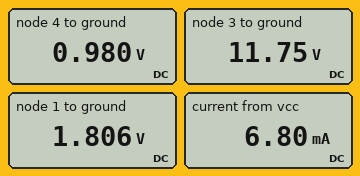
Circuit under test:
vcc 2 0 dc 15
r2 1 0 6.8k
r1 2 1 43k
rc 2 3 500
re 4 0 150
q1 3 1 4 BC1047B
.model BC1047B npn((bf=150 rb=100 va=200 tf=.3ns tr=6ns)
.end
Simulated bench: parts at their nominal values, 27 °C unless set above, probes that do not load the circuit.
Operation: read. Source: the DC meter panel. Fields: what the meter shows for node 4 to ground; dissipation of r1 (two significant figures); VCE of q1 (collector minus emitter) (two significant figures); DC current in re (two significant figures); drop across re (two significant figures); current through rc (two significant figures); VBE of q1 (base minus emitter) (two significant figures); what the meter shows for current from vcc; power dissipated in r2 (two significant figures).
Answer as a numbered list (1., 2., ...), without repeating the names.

1. 0.980 V
2. 4.0 mW
3. 11 V
4. 6.5 mA
5. 980 mV
6. 6.5 mA
7. 830 mV
8. 6.80 mA
9. 480 µW
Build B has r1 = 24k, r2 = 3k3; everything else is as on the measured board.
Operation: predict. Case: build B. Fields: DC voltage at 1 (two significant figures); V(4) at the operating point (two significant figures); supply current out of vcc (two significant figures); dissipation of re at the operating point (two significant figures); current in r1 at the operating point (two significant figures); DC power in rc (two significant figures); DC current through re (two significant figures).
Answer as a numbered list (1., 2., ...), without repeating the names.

1. 1.7 V
2. 880 mV
3. 6.4 mA
4. 5.2 mW
5. 550 µA
6. 17 mW
7. 5.9 mA
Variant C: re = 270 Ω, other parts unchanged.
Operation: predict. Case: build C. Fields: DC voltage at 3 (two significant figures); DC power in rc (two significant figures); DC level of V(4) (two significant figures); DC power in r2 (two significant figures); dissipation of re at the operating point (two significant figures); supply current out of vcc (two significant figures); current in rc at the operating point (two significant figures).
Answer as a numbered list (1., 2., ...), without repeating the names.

1. 13 V
2. 8.0 mW
3. 1.1 V
4. 530 µW
5. 4.4 mW
6. 4.3 mA
7. 4.0 mA
